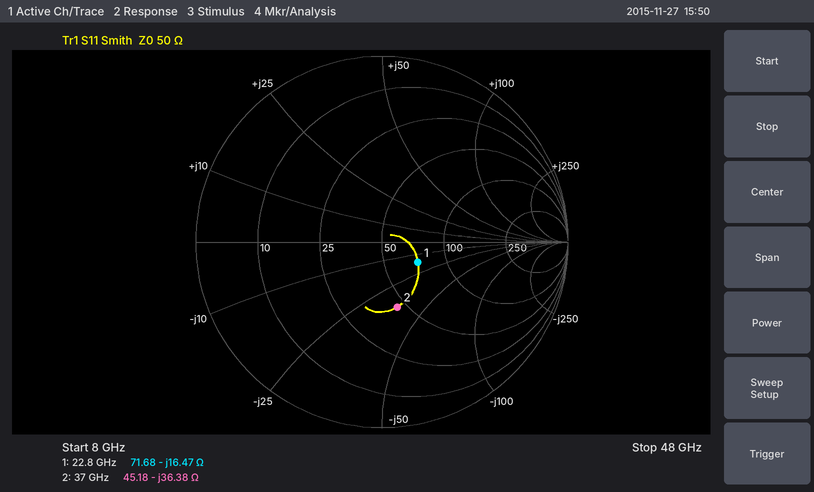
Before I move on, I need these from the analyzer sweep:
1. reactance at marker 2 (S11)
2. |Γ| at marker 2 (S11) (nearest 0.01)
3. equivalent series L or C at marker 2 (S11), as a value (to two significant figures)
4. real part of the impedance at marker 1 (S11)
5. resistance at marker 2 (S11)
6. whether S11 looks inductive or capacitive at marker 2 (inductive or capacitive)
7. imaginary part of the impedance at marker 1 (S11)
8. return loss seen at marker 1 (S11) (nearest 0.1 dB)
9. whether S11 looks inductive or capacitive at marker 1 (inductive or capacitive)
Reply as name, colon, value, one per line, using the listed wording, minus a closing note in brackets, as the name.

reactance at marker 2: -36.38 Ω
|Γ| at marker 2 (S11): 0.36
equivalent series L or C at marker 2 (S11), as a value: 120 fF
real part of the impedance at marker 1: 71.68 Ω
resistance at marker 2: 45.18 Ω
whether S11 looks inductive or capacitive at marker 2: capacitive
imaginary part of the impedance at marker 1: -16.47 Ω
return loss seen at marker 1 (S11): 13.1 dB
whether S11 looks inductive or capacitive at marker 1: capacitive
